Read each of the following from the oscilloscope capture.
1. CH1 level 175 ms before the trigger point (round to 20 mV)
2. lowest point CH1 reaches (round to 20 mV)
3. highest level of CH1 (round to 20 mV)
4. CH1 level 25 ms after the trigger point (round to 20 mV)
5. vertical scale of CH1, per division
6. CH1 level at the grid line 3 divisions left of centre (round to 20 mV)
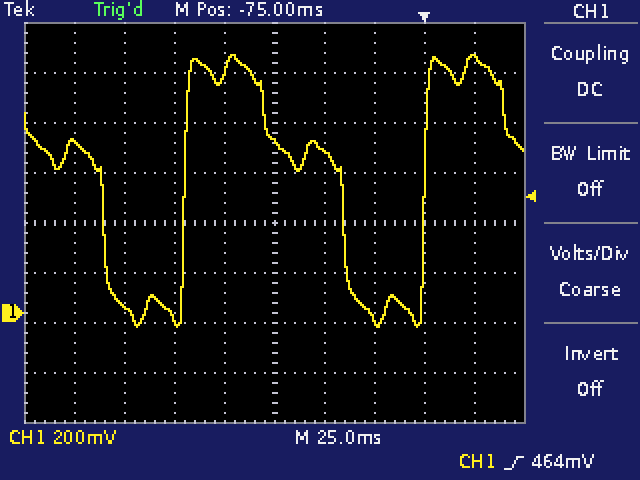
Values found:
680 mV
-60 mV
1.04 V
1.02 V
200 mV
20 mV
